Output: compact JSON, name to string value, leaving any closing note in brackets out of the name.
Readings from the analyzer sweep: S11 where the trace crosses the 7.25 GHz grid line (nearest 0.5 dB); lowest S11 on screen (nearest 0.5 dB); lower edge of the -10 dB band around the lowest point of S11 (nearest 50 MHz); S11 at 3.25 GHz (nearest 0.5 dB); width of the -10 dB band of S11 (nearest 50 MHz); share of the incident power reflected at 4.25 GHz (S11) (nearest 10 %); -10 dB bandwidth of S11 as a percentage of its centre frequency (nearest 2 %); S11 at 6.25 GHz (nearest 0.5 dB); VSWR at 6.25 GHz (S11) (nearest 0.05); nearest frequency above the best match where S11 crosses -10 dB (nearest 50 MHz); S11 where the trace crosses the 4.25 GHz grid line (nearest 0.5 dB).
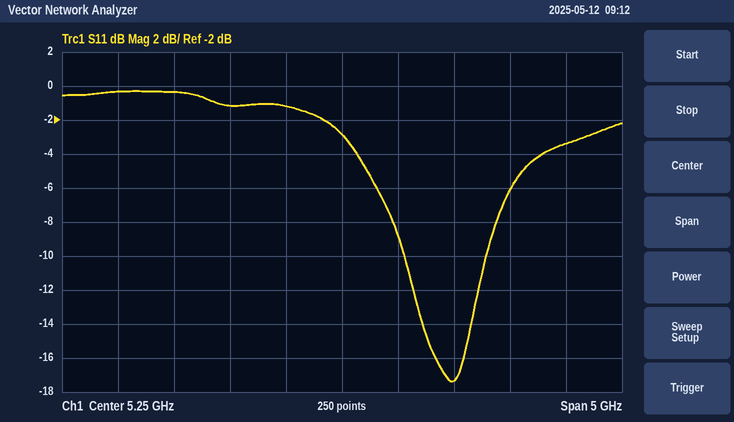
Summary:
{"S11 where the trace crosses the 7.25 GHz grid line": "-3.5 dB", "lowest S11 on screen": "-17.5 dB", "lower edge of the -10 dB band around the lowest point of S11": "5.80 GHz", "S11 at 3.25 GHz": "-0.5 dB", "width of the -10 dB band of S11": "750 MHz", "share of the incident power reflected at 4.25 GHz (S11)": "80 %", "-10 dB bandwidth of S11 as a percentage of its centre frequency": "12 %", "S11 at 6.25 GHz": "-17.5 dB", "VSWR at 6.25 GHz (S11)": "1.30", "nearest frequency above the best match where S11 crosses -10 dB": "6.55 GHz", "S11 where the trace crosses the 4.25 GHz grid line": "-1.0 dB"}
